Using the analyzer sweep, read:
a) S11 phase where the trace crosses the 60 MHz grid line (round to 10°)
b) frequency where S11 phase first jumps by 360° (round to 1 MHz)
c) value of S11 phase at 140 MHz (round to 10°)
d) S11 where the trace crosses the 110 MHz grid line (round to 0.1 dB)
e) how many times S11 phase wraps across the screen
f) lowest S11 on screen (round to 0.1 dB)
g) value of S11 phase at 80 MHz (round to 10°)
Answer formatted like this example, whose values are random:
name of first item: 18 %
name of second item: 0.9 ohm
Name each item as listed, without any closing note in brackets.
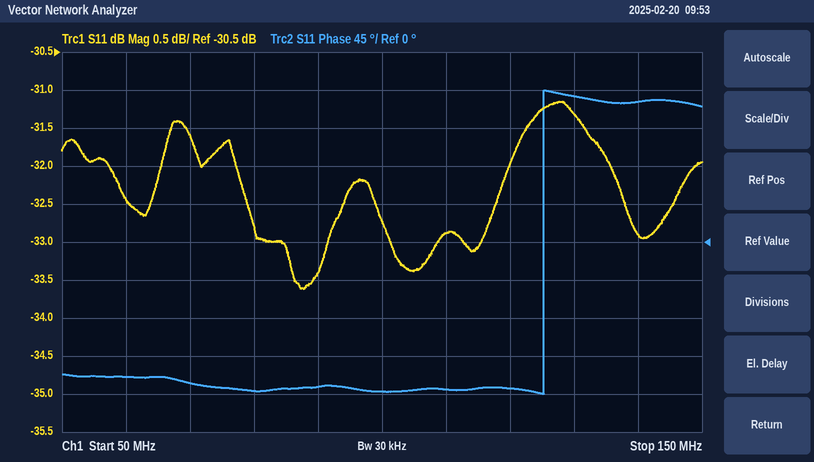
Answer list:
S11 phase where the trace crosses the 60 MHz grid line: -160°
frequency where S11 phase first jumps by 360°: 125 MHz
value of S11 phase at 140 MHz: 170°
S11 where the trace crosses the 110 MHz grid line: -32.9 dB
how many times S11 phase wraps across the screen: 1
lowest S11 on screen: -33.6 dB
value of S11 phase at 80 MHz: -180°
